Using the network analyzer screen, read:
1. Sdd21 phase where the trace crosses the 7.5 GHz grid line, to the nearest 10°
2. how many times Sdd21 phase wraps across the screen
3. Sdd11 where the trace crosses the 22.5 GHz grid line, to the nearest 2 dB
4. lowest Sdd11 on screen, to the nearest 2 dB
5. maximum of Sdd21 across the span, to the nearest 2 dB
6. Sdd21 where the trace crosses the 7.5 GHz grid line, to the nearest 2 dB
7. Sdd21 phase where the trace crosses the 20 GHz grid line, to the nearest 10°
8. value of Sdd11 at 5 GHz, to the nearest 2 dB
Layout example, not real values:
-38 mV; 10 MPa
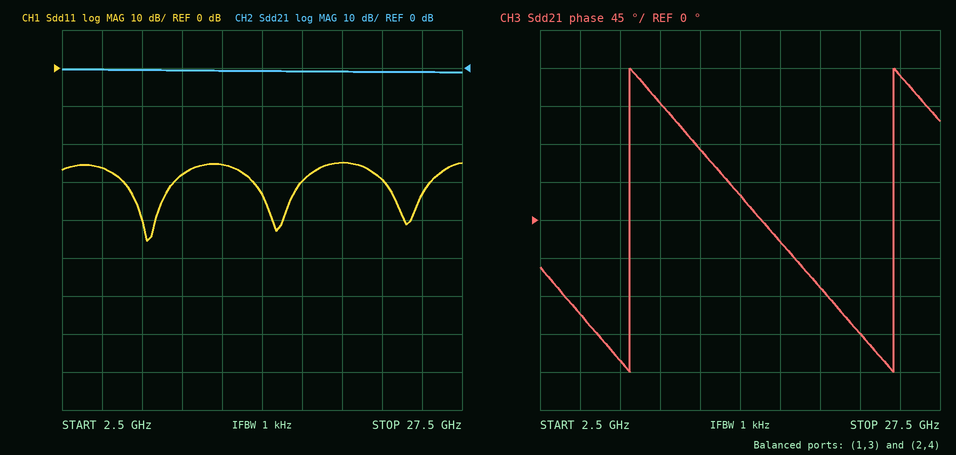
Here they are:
-170°; 2; -30 dB; -46 dB; 0 dB; 0 dB; -80°; -26 dB
